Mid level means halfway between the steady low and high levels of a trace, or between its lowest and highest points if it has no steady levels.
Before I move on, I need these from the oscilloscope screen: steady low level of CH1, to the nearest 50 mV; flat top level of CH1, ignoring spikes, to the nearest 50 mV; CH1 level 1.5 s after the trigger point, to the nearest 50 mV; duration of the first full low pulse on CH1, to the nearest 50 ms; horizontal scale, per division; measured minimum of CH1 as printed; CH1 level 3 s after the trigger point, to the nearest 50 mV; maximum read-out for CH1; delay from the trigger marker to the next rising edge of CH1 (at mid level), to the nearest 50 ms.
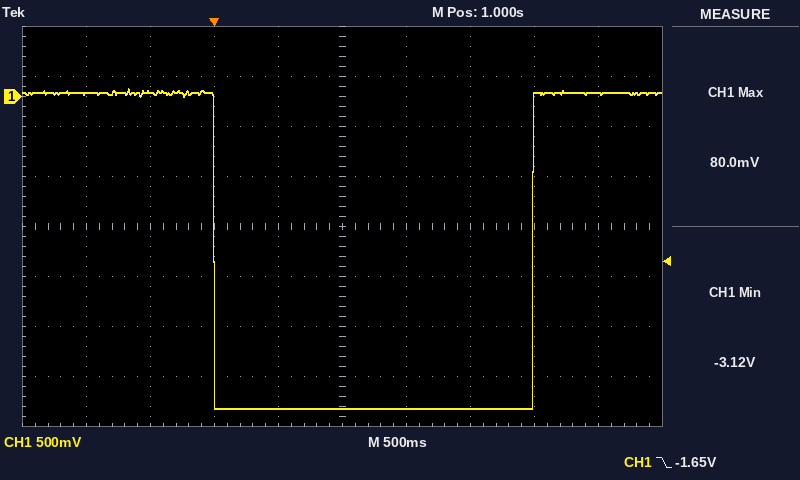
-3.10 V
50 mV
-3.10 V
2.50 s
500 ms
-3.12 V
50 mV
80.0 mV
2.50 s
